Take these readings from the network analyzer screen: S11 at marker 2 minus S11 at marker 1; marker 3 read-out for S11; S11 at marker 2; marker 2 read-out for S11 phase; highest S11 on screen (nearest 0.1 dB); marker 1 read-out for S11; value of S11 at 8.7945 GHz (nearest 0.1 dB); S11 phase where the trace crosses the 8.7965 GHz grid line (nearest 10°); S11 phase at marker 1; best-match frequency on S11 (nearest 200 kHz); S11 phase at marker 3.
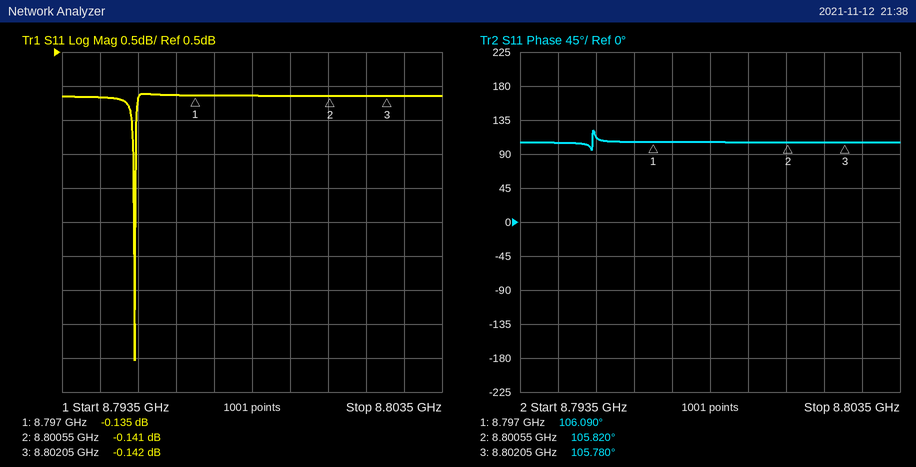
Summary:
-0.006 dB
-0.142 dB
-0.141 dB
105.820°
-0.1 dB
-0.135 dB
-0.2 dB
110°
106.090°
8.7954 GHz
105.780°
